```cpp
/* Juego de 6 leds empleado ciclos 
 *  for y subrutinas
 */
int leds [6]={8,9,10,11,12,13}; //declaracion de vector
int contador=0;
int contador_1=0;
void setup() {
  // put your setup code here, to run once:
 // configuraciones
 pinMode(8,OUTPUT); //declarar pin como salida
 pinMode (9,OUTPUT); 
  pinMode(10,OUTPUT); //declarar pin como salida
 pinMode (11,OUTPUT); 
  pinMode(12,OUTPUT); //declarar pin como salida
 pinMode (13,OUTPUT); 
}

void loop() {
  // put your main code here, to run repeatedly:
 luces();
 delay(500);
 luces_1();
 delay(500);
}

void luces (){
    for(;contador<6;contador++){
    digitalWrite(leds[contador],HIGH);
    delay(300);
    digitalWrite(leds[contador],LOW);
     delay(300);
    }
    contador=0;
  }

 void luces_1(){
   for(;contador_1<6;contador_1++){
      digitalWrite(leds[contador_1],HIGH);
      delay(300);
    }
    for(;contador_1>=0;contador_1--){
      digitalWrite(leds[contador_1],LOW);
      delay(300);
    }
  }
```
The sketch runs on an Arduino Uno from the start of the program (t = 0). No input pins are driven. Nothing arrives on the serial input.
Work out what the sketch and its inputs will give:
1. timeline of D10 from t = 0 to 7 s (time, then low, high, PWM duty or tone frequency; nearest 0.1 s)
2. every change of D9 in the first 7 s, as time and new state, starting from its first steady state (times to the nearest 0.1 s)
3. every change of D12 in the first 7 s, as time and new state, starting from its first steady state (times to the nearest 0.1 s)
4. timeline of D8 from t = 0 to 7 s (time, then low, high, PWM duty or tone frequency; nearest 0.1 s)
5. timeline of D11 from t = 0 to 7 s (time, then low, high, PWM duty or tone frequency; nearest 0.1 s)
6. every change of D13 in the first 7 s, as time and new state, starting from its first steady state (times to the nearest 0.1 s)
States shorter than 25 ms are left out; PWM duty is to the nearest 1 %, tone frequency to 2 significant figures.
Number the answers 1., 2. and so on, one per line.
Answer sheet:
1. 0 s low; 1.2 s high; 1.5 s low; 4.7 s high
2. 0 s low; 0.6 s high; 0.9 s low; 4.4 s high
3. 0 s low; 2.4 s high; 2.7 s low; 5.3 s high; 6.5 s low
4. 0 s high; 0.3 s low; 4.1 s high
5. 0 s low; 1.8 s high; 2.1 s low; 5 s high; 6.8 s low
6. 0 s low; 3 s high; 3.3 s low; 5.6 s high; 6.2 s low
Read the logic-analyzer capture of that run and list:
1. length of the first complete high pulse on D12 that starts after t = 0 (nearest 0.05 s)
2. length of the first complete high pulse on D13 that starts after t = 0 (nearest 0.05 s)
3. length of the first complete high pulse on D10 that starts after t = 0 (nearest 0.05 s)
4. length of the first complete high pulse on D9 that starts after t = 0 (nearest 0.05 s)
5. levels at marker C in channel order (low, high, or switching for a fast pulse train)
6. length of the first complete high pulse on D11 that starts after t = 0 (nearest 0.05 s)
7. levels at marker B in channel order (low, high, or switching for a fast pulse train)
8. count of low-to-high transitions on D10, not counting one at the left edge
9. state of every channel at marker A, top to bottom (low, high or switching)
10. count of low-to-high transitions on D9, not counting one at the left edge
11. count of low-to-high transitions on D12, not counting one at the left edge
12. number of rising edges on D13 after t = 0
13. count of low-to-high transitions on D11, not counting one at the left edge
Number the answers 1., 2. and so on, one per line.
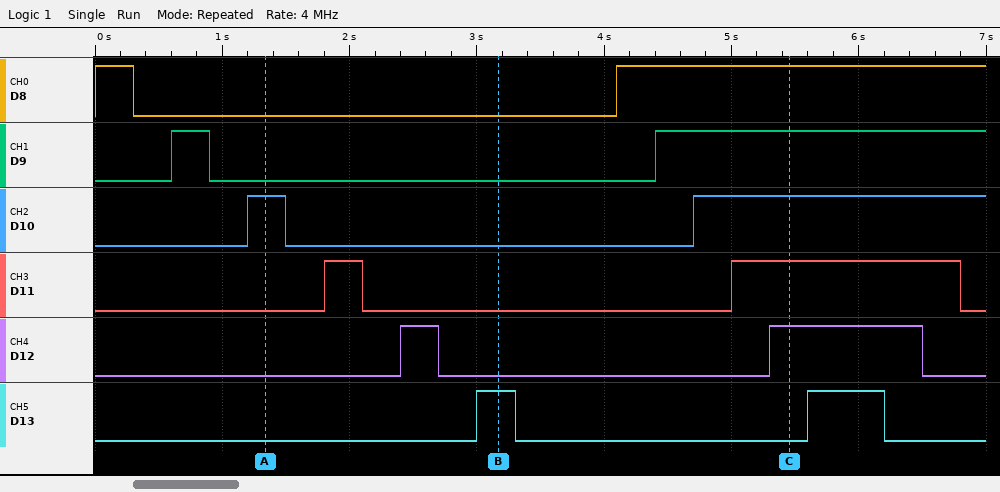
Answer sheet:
1. 0.30 s
2. 0.30 s
3. 0.30 s
4. 0.30 s
5. D8 high, D9 high, D10 high, D11 high, D12 high, D13 low
6. 0.30 s
7. D8 low, D9 low, D10 low, D11 low, D12 low, D13 high
8. 2
9. D8 low, D9 low, D10 high, D11 low, D12 low, D13 low
10. 2
11. 2
12. 2
13. 2
